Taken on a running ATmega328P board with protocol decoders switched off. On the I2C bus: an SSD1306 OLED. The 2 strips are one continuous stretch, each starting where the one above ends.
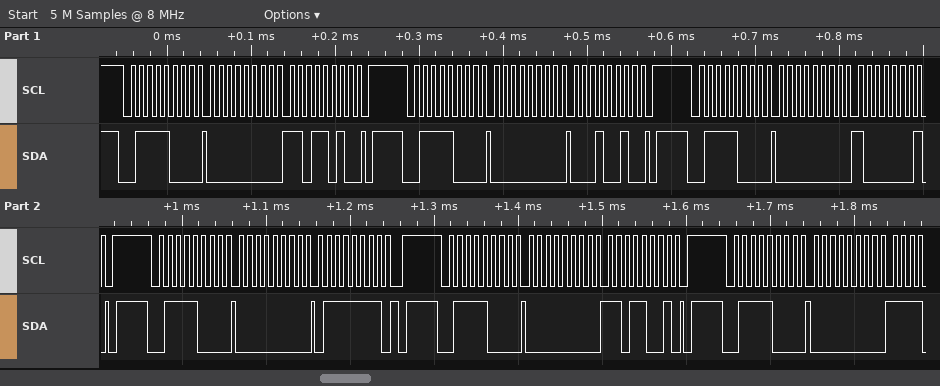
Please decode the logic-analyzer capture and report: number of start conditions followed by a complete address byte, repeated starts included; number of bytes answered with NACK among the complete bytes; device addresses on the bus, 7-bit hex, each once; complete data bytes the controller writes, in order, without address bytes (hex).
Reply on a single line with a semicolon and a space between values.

6; 0; 0x3C; 00 DA 00 12 00 81 00 7F 00 D9 00
